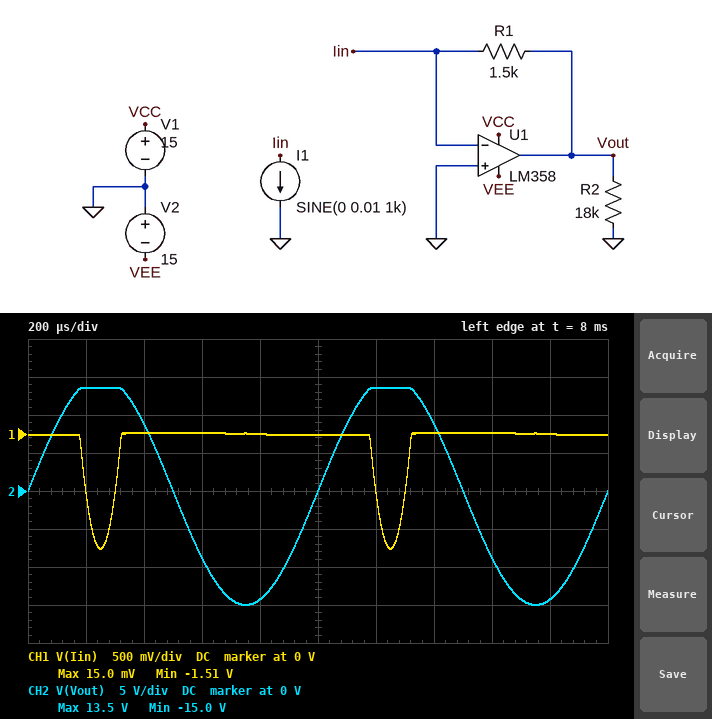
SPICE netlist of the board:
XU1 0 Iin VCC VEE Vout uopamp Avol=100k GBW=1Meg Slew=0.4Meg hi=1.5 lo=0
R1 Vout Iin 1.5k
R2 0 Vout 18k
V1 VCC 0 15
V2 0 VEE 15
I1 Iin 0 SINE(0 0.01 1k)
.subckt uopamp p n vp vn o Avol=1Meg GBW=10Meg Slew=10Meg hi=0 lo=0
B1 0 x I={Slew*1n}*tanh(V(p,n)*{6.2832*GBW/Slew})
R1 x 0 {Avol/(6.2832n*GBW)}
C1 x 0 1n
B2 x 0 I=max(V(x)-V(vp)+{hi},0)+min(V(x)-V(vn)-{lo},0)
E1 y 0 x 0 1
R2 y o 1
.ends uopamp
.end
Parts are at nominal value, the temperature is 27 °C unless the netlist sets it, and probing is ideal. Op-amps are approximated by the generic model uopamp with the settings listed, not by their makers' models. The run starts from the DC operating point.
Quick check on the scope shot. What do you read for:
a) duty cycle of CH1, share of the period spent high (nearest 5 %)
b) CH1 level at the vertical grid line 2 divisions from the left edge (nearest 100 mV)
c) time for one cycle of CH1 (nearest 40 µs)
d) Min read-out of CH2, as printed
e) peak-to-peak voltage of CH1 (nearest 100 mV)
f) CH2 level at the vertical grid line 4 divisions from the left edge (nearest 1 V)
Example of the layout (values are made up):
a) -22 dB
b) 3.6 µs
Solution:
a) 90 %
b) 0 V
c) 1.00 ms
d) -15.0 V
e) 1.5 V
f) -14 V
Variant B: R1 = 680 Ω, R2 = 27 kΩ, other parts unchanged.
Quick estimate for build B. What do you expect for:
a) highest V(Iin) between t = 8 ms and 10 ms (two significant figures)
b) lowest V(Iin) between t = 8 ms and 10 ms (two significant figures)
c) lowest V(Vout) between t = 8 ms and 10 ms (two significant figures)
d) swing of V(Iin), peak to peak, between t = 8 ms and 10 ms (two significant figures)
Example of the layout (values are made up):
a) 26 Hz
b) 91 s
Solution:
a) 6.8 mV
b) -6.8 mV
c) -6.8 V
d) 14 mV
